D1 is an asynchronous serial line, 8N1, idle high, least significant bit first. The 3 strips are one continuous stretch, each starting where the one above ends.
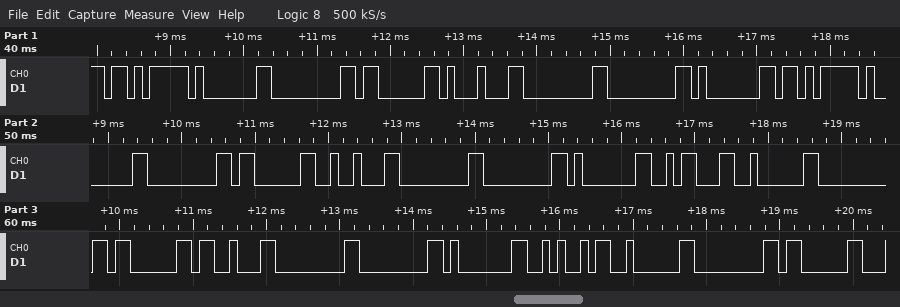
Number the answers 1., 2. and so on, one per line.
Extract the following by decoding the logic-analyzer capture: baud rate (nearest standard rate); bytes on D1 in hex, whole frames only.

1. 9600 baud
2. 0xEB 0x01 0x00 0x03 0x11 0x00 0x00 0x01 0xEB 0x01 0x00 0x03 0x12 0x00 0x00 0x01 0x1A 0x02 0x00 0x03 0x13 0x00 0x00 0x01 0x4A 0x02 0x00 0x03
